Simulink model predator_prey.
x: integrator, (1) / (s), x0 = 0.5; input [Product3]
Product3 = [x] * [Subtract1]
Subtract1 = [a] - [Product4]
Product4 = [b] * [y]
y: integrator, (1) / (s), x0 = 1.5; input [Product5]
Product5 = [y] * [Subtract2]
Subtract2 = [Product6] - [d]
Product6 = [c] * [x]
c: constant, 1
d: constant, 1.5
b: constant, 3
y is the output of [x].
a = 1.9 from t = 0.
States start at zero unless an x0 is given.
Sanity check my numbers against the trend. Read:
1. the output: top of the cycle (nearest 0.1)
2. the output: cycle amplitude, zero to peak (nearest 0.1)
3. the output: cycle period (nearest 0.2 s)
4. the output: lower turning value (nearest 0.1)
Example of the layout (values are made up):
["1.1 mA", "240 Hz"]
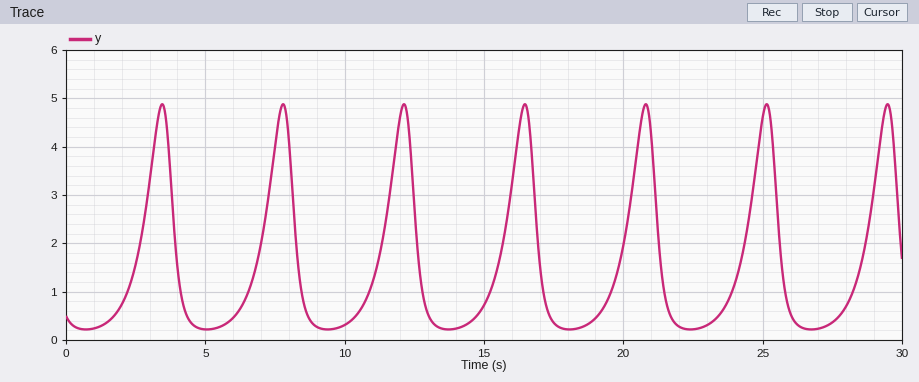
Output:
["4.9", "2.3", "4.4 s", "0.2"]
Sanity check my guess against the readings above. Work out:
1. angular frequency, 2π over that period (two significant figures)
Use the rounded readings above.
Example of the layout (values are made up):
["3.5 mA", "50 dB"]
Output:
["1.4 rad/s"]
